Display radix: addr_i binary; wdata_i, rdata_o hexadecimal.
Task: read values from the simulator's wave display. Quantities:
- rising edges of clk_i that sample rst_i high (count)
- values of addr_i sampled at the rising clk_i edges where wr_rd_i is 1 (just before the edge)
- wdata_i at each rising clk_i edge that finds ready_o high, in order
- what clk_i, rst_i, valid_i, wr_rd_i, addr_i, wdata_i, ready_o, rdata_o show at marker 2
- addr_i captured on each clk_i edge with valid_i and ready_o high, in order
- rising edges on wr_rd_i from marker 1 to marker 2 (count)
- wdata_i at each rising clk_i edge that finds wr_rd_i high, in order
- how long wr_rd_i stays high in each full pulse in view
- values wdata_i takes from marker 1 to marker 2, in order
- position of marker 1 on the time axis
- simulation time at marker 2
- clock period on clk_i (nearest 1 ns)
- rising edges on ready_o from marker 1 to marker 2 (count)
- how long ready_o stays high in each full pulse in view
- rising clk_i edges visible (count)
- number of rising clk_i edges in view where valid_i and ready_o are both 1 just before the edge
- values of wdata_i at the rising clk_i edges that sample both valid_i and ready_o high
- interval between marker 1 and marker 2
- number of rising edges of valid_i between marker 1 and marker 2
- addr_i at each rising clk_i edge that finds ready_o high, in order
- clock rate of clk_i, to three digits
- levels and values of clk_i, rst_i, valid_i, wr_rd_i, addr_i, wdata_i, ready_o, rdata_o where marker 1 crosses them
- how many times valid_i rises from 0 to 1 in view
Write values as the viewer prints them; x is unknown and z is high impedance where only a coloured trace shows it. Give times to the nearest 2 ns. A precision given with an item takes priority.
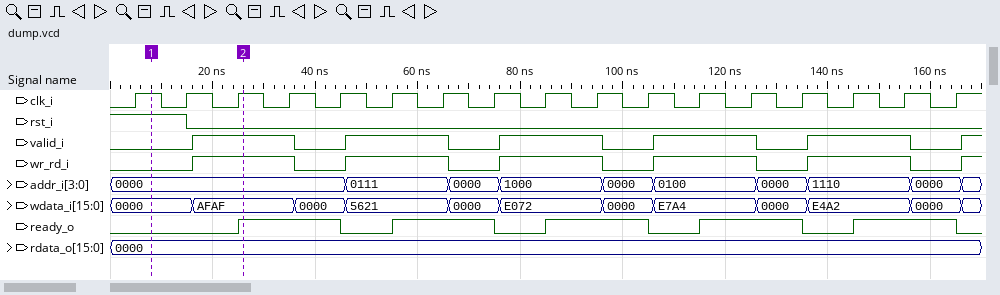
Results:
2
0000, 0000, 0111, 0111, 1000, 1000, 0100, 0100, 1110, 1110
AFAF, 0000, 5621, 0000, E072, 0000, E7A4, 0000, E4A2, 0000
clk_i=1, rst_i=0, valid_i=1, wr_rd_i=1, addr_i=0000, wdata_i=AFAF, ready_o=1, rdata_o=0000
0000, 0111, 1000, 0100, 1110
1
AFAF, AFAF, 5621, 5621, E072, E072, E7A4, E7A4, E4A2, E4A2
20 ns, 20 ns, 20 ns, 20 ns, 20 ns
0000, AFAF
8 ns
26 ns
10 ns
1
20 ns, 20 ns, 20 ns, 20 ns, 20 ns
17
5
AFAF, 5621, E072, E7A4, E4A2
18 ns
1
0000, 0000, 0111, 0000, 1000, 0000, 0100, 0000, 1110, 0000
100 MHz
clk_i=1, rst_i=1, valid_i=0, wr_rd_i=0, addr_i=0000, wdata_i=0000, ready_o=0, rdata_o=0000
6
